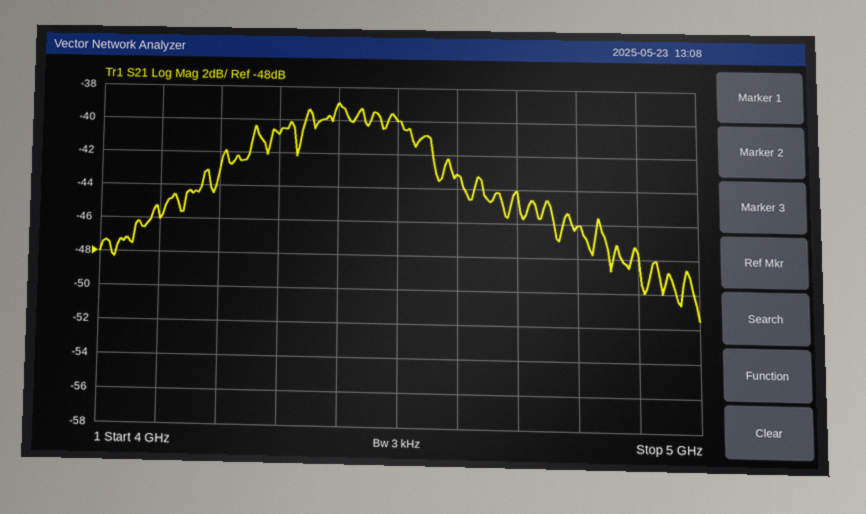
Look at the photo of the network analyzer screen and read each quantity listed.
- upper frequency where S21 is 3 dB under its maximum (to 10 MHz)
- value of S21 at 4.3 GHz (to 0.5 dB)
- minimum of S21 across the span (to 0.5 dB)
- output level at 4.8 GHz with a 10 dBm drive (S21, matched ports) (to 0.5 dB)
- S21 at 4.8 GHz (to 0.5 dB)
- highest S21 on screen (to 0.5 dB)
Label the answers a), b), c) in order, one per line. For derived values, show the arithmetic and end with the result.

a) 4.56 GHz
b) -41.0 dB
c) -51.5 dB
d) 10 dBm + (-46.0 dB) = -36.0 dBm
e) -46.0 dB
f) -39.0 dB
